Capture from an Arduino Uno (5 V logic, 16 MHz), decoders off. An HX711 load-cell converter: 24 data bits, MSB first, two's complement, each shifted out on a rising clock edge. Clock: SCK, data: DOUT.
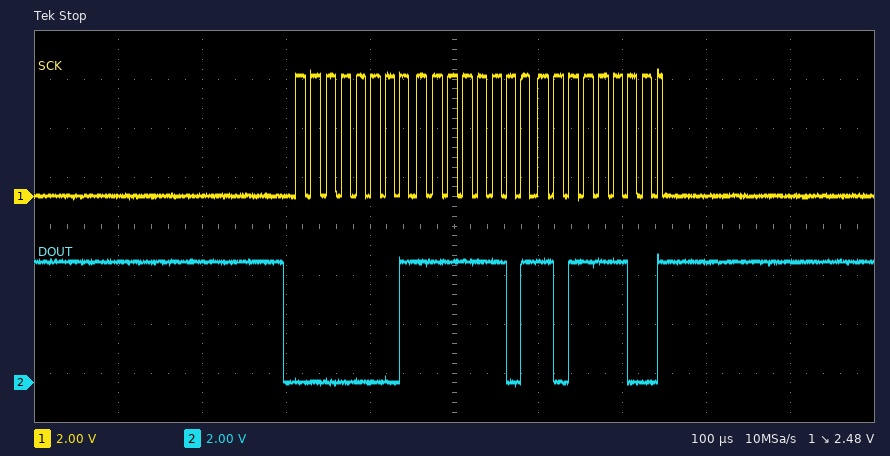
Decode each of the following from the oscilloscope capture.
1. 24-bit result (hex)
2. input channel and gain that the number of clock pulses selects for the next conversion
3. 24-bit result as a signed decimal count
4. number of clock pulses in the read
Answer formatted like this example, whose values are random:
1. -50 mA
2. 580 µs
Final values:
1. 0x01FDBC
2. channel A, gain 128
3. 130492
4. 25
